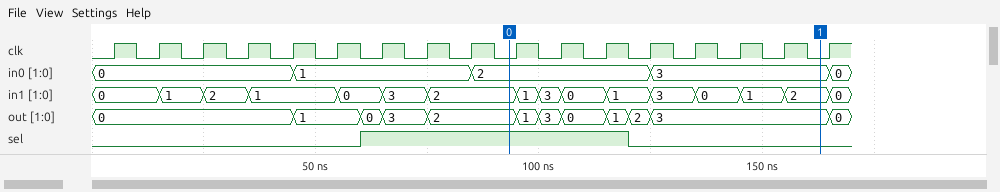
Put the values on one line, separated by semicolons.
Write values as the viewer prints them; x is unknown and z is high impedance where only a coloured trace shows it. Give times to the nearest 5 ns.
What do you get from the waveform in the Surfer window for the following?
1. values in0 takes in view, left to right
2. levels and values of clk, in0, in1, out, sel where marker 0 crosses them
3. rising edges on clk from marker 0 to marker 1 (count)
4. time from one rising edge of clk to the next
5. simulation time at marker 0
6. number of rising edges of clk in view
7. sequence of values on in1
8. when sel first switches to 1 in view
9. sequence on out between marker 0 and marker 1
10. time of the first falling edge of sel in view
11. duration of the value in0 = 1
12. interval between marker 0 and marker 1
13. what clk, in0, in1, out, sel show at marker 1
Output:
0, 1, 2, 3, 0; clk=0, in0=2, in1=2, out=2, sel=1; 7; 10 ns; 95 ns; 17; 0, 1, 2, 1, 0, 3, 2, 1, 3, 0, 1, 3, 0, 1, 2, 0; 60 ns; 2, 1, 3, 0, 1, 2, 3; 120 ns; 40 ns; 70 ns; clk=0, in0=3, in1=2, out=3, sel=0
